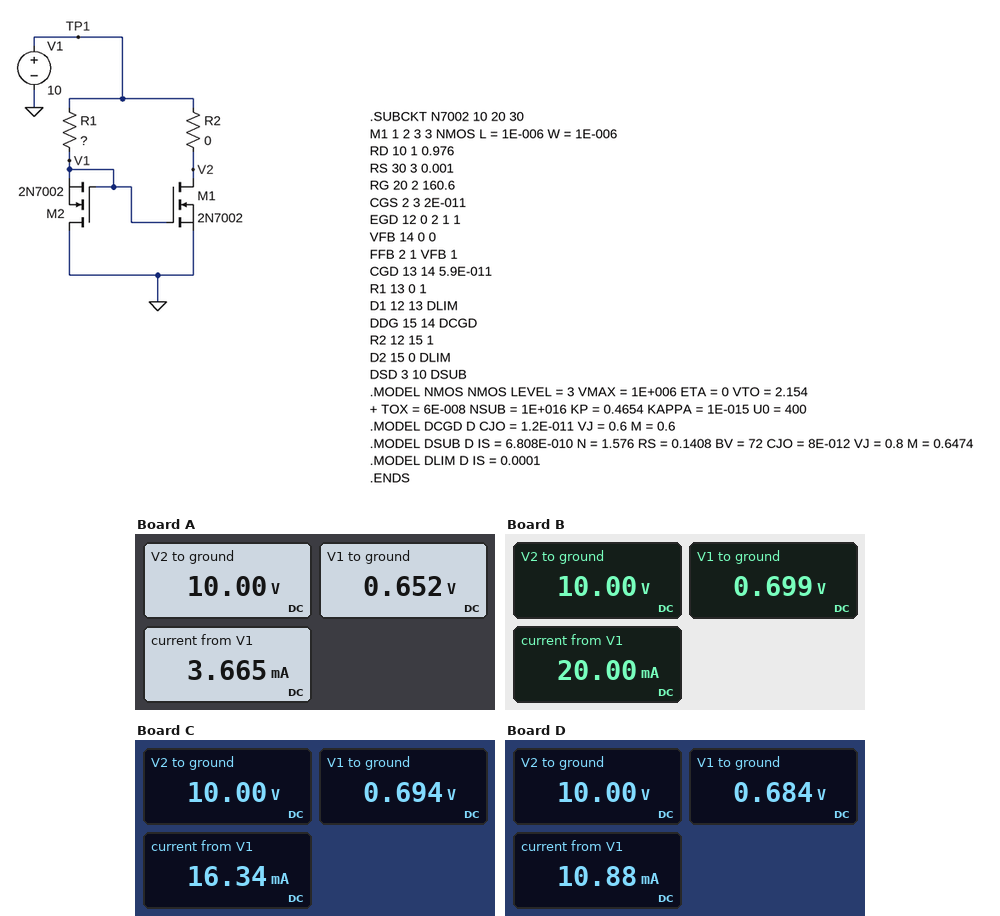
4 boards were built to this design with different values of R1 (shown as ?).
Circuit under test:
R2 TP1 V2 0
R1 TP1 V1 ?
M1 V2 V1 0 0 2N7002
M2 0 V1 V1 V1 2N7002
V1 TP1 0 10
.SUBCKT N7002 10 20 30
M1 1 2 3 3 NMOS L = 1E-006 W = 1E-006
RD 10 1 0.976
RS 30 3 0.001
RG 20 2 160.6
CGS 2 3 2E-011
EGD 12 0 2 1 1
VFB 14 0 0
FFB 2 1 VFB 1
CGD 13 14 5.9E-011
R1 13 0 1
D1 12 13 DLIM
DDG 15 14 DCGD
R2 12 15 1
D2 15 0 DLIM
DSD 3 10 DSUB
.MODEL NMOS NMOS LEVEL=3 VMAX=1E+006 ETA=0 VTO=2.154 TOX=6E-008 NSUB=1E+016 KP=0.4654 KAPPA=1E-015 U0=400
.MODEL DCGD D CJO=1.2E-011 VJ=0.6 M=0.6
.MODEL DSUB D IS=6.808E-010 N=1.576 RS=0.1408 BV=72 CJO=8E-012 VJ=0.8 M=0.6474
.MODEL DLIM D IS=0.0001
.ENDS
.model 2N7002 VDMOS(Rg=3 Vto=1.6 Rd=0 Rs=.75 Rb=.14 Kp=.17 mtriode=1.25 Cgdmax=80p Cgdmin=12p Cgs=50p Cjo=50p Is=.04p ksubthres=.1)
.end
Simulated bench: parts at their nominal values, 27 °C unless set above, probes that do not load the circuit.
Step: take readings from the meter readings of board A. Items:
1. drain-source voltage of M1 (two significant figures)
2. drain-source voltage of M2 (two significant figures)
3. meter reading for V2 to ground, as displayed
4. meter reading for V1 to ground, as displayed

10 V
-650 mV
10.00 V
0.652 V
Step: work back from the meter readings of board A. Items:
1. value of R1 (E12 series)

2.7 kΩ
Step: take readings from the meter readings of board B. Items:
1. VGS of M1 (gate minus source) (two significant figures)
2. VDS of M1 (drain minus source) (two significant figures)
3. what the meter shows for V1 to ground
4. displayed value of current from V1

700 mV
10 V
0.699 V
20.00 mA
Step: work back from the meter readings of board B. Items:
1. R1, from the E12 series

470 Ω
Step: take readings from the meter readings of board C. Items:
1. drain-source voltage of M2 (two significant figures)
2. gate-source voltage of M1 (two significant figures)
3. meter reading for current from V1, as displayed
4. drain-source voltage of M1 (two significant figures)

-690 mV
690 mV
16.34 mA
10 V
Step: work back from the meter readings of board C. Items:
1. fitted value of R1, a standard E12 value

560 Ω
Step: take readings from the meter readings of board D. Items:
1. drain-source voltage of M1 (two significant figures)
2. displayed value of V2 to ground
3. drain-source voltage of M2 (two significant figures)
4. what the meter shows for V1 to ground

10 V
10.00 V
-680 mV
0.684 V
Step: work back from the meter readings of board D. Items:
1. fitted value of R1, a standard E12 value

820 Ω
